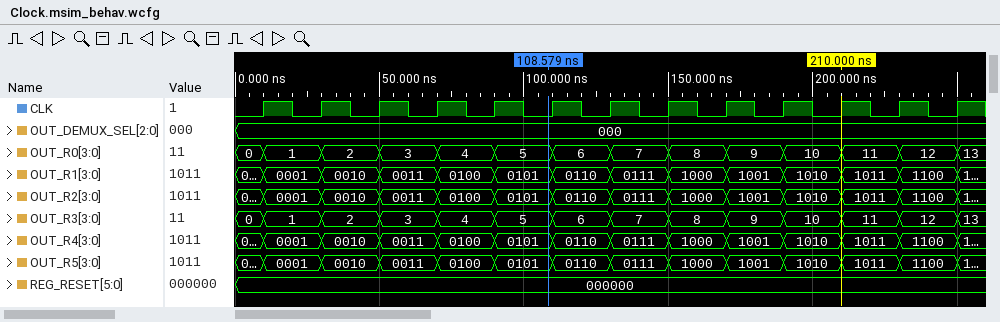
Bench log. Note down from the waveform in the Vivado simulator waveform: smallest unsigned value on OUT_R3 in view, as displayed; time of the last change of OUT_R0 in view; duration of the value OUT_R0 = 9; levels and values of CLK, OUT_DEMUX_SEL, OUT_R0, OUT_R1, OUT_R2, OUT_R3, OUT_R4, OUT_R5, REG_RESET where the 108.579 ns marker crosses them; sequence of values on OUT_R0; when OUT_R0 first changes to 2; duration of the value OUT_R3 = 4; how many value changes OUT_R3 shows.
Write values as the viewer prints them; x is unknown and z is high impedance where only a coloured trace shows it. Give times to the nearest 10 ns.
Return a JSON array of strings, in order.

["0", "250 ns", "20 ns", "CLK=0, OUT_DEMUX_SEL=000, OUT_R0=5, OUT_R1=0101, OUT_R2=0101, OUT_R3=5, OUT_R4=0101, OUT_R5=0101, REG_RESET=000000", "0, 1, 2, 3, 4, 5, 6, 7, 8, 9, 10, 11, 12, 13", "30 ns", "20 ns", "13"]
